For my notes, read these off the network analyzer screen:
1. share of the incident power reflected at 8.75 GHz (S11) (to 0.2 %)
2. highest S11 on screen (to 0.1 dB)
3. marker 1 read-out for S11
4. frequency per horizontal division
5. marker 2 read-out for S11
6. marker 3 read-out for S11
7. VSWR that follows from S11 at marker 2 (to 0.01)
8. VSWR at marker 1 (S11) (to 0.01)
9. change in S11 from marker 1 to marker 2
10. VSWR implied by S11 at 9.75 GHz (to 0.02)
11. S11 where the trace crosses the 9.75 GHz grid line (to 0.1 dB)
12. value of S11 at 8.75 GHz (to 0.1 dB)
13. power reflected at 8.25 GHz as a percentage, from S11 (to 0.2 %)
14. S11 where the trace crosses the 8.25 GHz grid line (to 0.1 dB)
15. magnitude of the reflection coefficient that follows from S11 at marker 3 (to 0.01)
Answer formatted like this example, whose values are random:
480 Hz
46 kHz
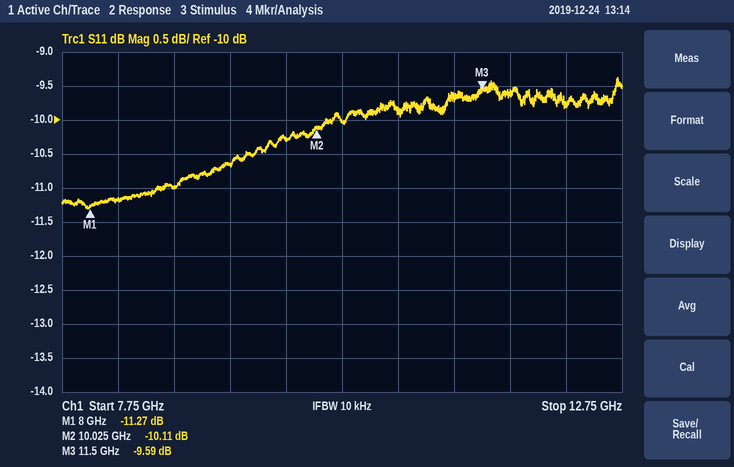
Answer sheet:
8.0 %
-9.4 dB
-11.27 dB
500 MHz
-10.11 dB
-9.59 dB
1.91
1.75
1.16 dB
1.88
-10.3 dB
-11.0 dB
7.6 %
-11.2 dB
0.33
